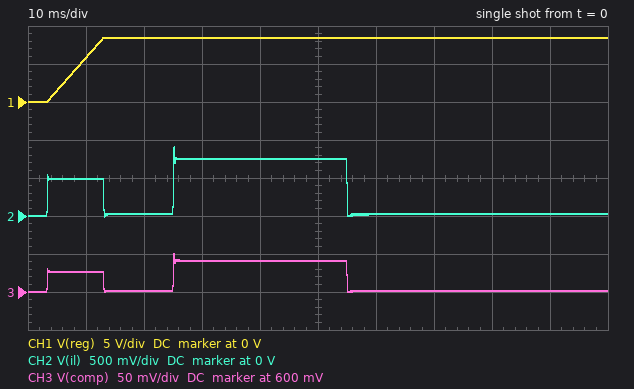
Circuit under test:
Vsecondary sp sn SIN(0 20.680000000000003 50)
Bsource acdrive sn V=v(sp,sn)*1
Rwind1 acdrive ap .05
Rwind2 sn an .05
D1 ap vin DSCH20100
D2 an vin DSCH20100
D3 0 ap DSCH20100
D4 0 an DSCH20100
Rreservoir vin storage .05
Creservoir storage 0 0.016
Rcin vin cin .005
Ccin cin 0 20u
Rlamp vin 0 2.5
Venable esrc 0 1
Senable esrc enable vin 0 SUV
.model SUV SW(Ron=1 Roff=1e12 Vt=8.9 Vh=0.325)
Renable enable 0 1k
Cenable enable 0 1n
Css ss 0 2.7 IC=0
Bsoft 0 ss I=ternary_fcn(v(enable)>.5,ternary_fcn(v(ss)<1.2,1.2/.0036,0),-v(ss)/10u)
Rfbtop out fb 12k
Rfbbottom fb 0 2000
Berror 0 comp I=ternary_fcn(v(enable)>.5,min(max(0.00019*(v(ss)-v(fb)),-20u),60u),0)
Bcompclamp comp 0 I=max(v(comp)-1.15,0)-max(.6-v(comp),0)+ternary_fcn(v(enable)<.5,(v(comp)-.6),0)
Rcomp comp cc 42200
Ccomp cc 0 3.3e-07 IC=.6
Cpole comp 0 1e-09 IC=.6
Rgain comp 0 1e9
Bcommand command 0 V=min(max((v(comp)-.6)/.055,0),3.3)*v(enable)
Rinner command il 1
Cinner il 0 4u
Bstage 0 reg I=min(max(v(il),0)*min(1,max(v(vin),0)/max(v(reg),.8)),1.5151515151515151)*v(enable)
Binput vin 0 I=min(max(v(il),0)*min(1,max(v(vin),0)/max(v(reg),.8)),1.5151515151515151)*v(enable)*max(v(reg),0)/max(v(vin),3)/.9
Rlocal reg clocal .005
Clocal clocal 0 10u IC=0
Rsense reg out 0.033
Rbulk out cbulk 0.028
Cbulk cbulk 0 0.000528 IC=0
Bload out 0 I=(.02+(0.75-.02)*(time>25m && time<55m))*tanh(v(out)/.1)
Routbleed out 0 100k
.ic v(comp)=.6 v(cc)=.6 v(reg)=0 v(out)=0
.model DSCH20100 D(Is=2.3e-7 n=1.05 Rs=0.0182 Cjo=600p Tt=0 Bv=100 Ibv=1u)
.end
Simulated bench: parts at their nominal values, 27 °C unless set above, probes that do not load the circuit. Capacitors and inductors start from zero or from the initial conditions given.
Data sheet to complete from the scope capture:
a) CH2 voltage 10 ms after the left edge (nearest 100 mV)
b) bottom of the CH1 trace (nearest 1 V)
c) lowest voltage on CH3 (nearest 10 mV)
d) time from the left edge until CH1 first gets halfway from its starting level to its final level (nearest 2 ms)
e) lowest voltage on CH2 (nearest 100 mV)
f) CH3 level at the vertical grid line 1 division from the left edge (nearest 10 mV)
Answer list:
500 mV
0 V
600 mV
8 ms
0 V
630 mV
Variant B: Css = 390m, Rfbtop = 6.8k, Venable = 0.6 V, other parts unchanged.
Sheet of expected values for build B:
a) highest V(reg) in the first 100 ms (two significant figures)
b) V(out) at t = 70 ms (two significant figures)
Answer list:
5.4 V
5.3 V
